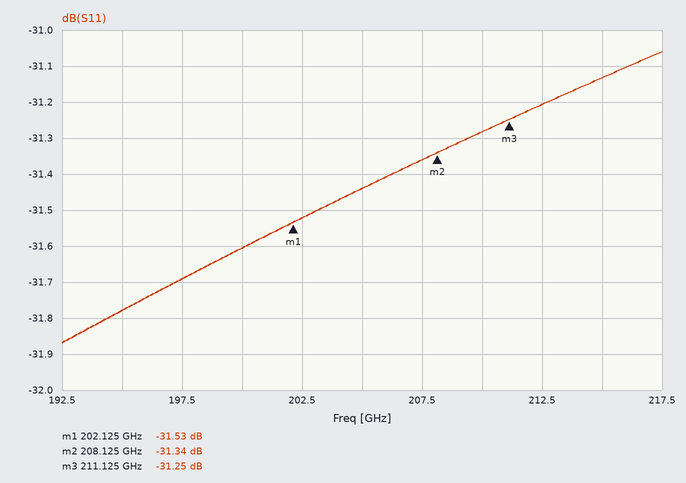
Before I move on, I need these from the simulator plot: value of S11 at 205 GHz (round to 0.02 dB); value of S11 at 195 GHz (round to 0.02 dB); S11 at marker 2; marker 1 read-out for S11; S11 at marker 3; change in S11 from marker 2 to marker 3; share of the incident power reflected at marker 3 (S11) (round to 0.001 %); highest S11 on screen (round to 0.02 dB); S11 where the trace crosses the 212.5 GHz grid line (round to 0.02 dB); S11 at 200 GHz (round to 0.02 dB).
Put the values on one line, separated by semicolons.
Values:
-31.44 dB; -31.78 dB; -31.34 dB; -31.53 dB; -31.25 dB; 0.09 dB; 0.075 %; -31.06 dB; -31.20 dB; -31.60 dB
